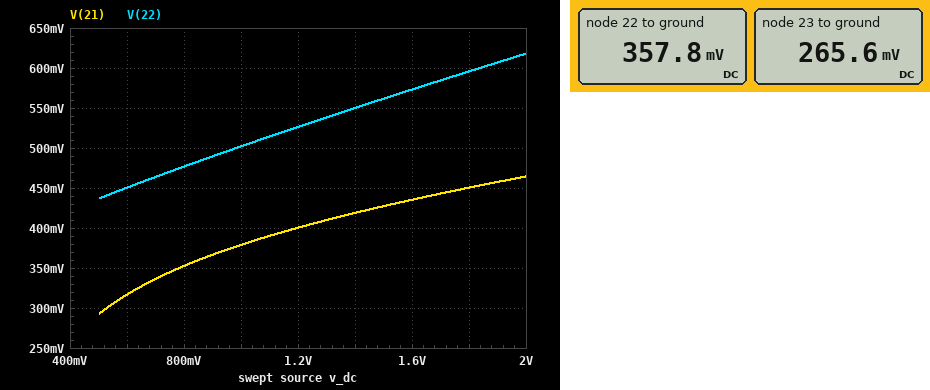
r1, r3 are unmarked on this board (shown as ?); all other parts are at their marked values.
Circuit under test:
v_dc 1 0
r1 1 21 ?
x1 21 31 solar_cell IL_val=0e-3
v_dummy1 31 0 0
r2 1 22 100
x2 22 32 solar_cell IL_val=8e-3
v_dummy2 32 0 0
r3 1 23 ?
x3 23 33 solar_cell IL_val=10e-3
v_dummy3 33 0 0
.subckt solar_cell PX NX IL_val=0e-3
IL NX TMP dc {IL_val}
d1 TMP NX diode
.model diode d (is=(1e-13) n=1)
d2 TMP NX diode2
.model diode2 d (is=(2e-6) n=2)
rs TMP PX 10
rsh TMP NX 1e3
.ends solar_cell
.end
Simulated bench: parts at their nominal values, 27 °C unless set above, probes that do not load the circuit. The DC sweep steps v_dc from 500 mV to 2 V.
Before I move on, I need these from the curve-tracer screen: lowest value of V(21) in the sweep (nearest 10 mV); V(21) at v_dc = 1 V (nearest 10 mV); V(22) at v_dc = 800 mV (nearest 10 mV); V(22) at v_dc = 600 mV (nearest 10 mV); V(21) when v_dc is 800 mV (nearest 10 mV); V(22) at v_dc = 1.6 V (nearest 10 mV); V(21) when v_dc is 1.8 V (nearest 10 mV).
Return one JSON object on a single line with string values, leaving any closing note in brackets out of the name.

{"lowest value of V(21) in the sweep": "290 mV", "V(21) at v_dc = 1 V": "380 mV", "V(22) at v_dc = 800 mV": "480 mV", "V(22) at v_dc = 600 mV": "450 mV", "V(21) when v_dc is 800 mV": "350 mV", "V(22) at v_dc = 1.6 V": "570 mV", "V(21) when v_dc is 1.8 V": "450 mV"}
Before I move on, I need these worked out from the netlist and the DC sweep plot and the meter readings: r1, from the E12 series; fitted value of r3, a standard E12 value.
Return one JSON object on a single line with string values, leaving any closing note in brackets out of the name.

{"r1, from the E12 series": "270 Ω", "fitted value of r3, a standard E12 value": "33 Ω"}
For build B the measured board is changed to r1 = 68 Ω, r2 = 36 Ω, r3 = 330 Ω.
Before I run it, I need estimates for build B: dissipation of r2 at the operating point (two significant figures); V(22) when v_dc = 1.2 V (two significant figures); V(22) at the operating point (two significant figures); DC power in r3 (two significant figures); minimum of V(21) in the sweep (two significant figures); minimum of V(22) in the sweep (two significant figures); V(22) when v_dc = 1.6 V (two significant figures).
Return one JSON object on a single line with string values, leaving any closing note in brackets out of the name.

{"dissipation of r2 at the operating point": "1.7 mW", "V(22) when v_dc = 1.2 V": "640 mV", "V(22) at the operating point": "250 mV", "DC power in r3": "530 µW", "minimum of V(21) in the sweep": "370 mV", "minimum of V(22) in the sweep": "450 mV", "V(22) when v_dc = 1.6 V": "740 mV"}
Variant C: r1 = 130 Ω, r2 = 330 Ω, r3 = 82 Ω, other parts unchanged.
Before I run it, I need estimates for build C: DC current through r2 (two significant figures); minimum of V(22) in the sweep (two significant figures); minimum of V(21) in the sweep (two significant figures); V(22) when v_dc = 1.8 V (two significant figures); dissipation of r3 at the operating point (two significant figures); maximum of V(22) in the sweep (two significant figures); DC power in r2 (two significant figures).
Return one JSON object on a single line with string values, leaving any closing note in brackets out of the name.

{"DC current through r2": "1.2 mA", "minimum of V(22) in the sweep": "430 mV", "minimum of V(21) in the sweep": "330 mV", "V(22) when v_dc = 1.8 V": "490 mV", "dissipation of r3 at the operating point": "1.6 mW", "maximum of V(22) in the sweep": "500 mV", "DC power in r2": "500 µW"}
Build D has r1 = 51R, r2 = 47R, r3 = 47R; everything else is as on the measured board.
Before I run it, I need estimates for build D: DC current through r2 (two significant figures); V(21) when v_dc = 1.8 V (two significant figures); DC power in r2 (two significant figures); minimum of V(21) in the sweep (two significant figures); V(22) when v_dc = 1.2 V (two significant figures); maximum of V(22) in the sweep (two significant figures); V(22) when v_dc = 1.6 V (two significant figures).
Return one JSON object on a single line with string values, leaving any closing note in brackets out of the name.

{"DC current through r2": "6.1 mA", "V(21) when v_dc = 1.8 V": "700 mV", "DC power in r2": "1.7 mW", "minimum of V(21) in the sweep": "380 mV", "V(22) when v_dc = 1.2 V": "600 mV", "maximum of V(22) in the sweep": "770 mV", "V(22) when v_dc = 1.6 V": "690 mV"}
